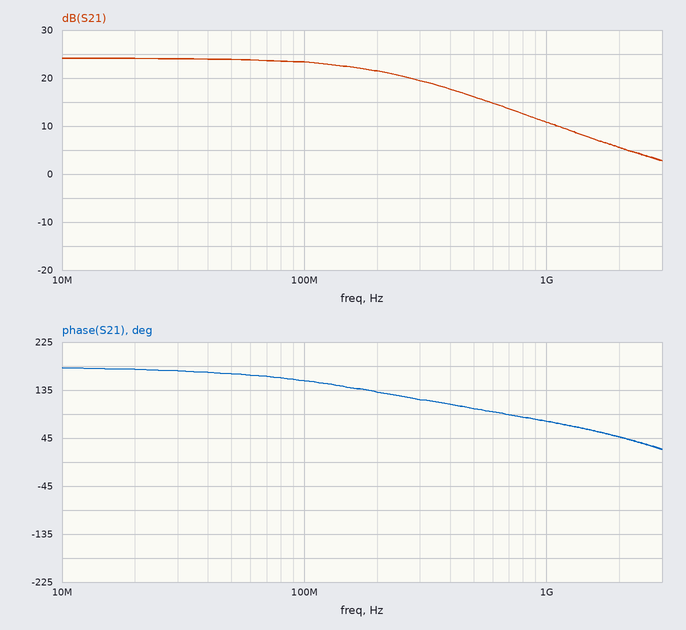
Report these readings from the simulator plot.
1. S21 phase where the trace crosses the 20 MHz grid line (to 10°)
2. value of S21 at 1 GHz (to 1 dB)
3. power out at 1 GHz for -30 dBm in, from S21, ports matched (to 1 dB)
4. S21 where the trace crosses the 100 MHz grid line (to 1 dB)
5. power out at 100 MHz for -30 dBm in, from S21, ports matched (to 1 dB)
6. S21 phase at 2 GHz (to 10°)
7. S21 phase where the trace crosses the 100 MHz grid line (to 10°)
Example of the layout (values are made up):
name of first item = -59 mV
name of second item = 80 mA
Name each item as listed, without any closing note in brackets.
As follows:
S21 phase where the trace crosses the 20 MHz grid line = 170°
value of S21 at 1 GHz = 11 dB
power out at 1 GHz for -30 dBm in, from S21, ports matched = -19 dBm
S21 where the trace crosses the 100 MHz grid line = 23 dB
power out at 100 MHz for -30 dBm in, from S21, ports matched = -7 dBm
S21 phase at 2 GHz = 50°
S21 phase where the trace crosses the 100 MHz grid line = 150°
